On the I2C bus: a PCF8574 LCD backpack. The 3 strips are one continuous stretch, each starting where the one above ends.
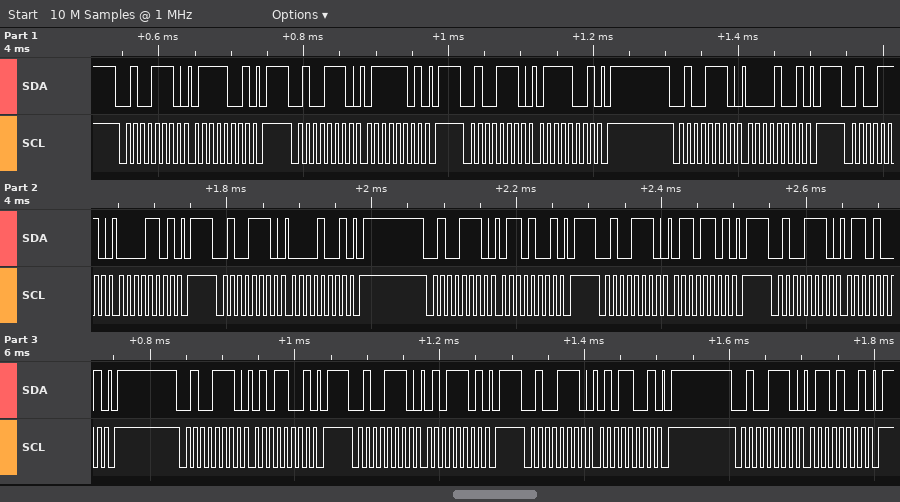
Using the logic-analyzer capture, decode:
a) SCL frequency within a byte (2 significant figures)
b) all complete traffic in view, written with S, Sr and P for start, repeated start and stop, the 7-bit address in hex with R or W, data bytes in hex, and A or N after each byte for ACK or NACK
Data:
100 kHz
S 27W A 79 A P S 27W A 7D A P S 27W A 79 A P S 27W A 09 A P S 27W A 0D A P S 27W A 09 A P S 27W A 69 A P S 27W A 6D A P S 27W A 69 A P S 27W A 59 A P S 27W A 5D A P S 27W A 59 A P S 27W A 69 A P
